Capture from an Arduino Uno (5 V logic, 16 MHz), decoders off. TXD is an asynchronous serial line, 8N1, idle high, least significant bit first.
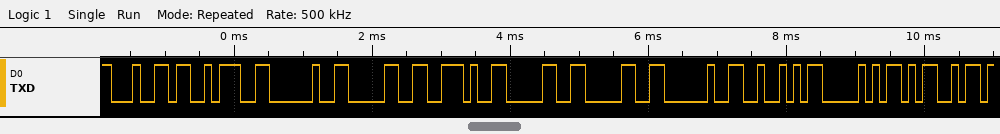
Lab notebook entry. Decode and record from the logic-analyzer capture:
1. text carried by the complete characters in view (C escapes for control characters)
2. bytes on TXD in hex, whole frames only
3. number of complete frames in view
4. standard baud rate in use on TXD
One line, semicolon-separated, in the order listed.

"d: 0.00 RPM"; 64 3A 20 30 2E 30 30 20 52 50 4D; 11; 9600 baud
